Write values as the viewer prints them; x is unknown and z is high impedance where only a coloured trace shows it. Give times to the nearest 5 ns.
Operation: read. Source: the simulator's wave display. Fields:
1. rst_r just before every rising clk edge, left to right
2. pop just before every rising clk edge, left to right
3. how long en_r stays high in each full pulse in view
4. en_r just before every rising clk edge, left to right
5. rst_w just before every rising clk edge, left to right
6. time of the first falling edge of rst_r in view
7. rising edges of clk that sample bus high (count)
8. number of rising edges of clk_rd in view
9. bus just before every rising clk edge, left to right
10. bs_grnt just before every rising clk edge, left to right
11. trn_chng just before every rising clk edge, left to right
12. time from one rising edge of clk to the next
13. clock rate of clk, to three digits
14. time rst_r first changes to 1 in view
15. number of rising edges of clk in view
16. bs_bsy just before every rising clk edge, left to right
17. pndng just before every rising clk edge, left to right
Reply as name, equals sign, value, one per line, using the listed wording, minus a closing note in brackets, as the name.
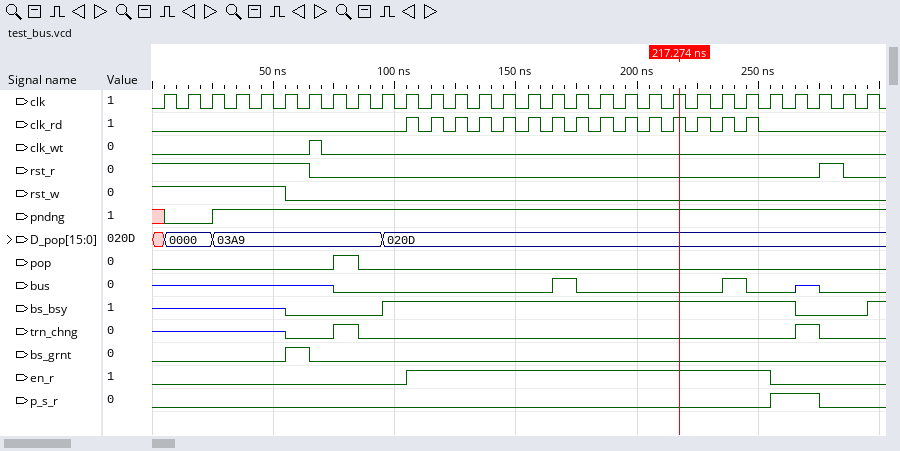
rst_r just before every rising clk edge, left to right = 1 1 1 1 1 1 1 0 0 0 0 0 0 0 0 0 0 0 0 0 0 0 0 0 0 0 0 0 1 0
pop just before every rising clk edge, left to right = 0 0 0 0 0 0 0 0 1 0 0 0 0 0 0 0 0 0 0 0 0 0 0 0 0 0 0 0 0 0
how long en_r stays high in each full pulse in view = 150 ns
en_r just before every rising clk edge, left to right = 0 0 0 0 0 0 0 0 0 0 0 1 1 1 1 1 1 1 1 1 1 1 1 1 1 1 0 0 0 0
rst_w just before every rising clk edge, left to right = 1 1 1 1 1 1 0 0 0 0 0 0 0 0 0 0 0 0 0 0 0 0 0 0 0 0 0 0 0 0
time of the first falling edge of rst_r in view = 65 ns
rising edges of clk that sample bus high = 2
number of rising edges of clk_rd in view = 15
bus just before every rising clk edge, left to right = z z z z z z z z 0 0 0 0 0 0 0 0 0 1 0 0 0 0 0 0 1 0 0 z 0 0
bs_grnt just before every rising clk edge, left to right = 0 0 0 0 0 0 1 0 0 0 0 0 0 0 0 0 0 0 0 0 0 0 0 0 0 0 0 0 0 0
trn_chng just before every rising clk edge, left to right = z z z z z z 0 0 1 0 0 0 0 0 0 0 0 0 0 0 0 0 0 0 0 0 0 1 0 0
time from one rising edge of clk to the next = 10 ns
clock rate of clk, to three digits = 100 MHz
time rst_r first changes to 1 in view = 275 ns
number of rising edges of clk in view = 30
bs_bsy just before every rising clk edge, left to right = z z z z z z 0 0 0 0 1 1 1 1 1 1 1 1 1 1 1 1 1 1 1 1 1 0 0 0
pndng just before every rising clk edge, left to right = x 0 0 1 1 1 1 1 1 1 1 1 1 1 1 1 1 1 1 1 1 1 1 1 1 1 1 1 1 1
